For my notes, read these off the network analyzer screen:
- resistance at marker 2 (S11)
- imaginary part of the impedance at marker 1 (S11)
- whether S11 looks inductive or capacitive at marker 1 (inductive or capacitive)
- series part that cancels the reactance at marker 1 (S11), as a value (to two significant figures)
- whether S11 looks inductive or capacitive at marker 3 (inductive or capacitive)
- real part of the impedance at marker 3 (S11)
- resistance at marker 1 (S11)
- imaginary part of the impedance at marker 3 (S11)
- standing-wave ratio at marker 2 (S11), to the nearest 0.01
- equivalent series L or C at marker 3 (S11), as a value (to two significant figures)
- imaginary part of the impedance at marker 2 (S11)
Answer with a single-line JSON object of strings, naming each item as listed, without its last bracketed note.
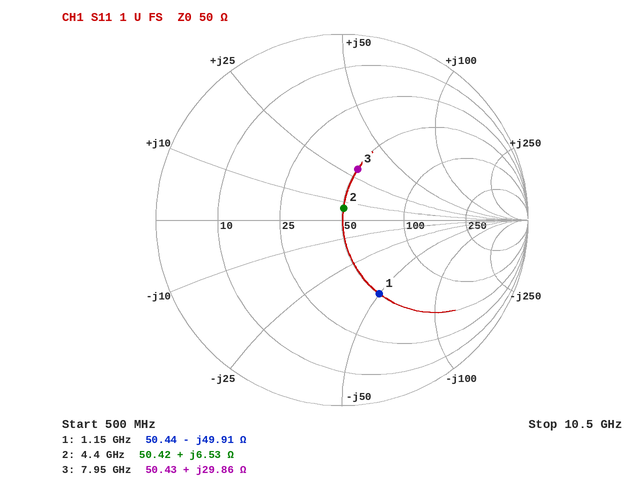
{"resistance at marker 2": "50.42 Ω", "imaginary part of the impedance at marker 1": "-49.91 Ω", "whether S11 looks inductive or capacitive at marker 1": "capacitive", "series part that cancels the reactance at marker 1 (S11), as a value": "6.9 nH", "whether S11 looks inductive or capacitive at marker 3": "inductive", "real part of the impedance at marker 3": "50.43 Ω", "resistance at marker 1": "50.44 Ω", "imaginary part of the impedance at marker 3": "+29.86 Ω", "standing-wave ratio at marker 2 (S11), to the nearest 0.01": "1.14", "equivalent series L or C at marker 3 (S11), as a value": "600 pH", "imaginary part of the impedance at marker 2": "+6.53 Ω"}
